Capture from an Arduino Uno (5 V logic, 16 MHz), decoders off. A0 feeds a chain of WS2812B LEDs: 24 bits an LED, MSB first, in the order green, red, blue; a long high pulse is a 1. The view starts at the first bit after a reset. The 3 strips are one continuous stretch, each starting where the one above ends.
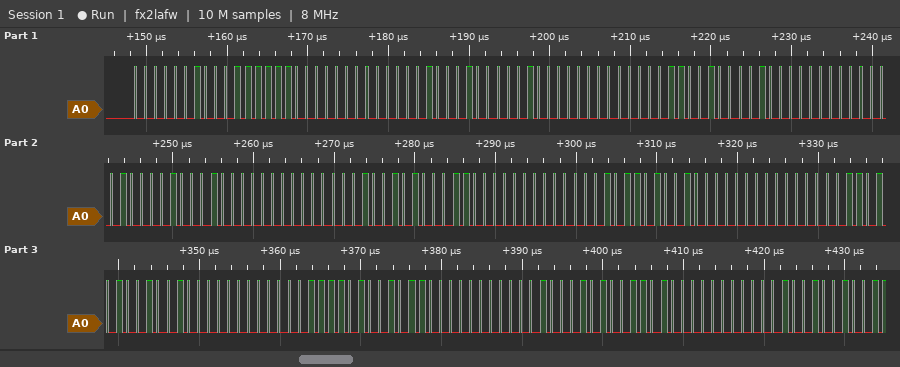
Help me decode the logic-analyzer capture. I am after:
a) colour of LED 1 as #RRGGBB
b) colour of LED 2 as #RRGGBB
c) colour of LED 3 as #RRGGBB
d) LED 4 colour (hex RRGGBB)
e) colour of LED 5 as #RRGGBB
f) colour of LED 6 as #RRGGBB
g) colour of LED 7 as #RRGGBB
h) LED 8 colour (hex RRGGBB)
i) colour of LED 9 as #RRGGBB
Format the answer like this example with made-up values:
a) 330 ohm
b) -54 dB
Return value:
a) #3F0200
b) #410400
c) #420600
d) #440800
e) #460900
f) #480B00
g) #490D00
h) #4B0F00
i) #4D1100
